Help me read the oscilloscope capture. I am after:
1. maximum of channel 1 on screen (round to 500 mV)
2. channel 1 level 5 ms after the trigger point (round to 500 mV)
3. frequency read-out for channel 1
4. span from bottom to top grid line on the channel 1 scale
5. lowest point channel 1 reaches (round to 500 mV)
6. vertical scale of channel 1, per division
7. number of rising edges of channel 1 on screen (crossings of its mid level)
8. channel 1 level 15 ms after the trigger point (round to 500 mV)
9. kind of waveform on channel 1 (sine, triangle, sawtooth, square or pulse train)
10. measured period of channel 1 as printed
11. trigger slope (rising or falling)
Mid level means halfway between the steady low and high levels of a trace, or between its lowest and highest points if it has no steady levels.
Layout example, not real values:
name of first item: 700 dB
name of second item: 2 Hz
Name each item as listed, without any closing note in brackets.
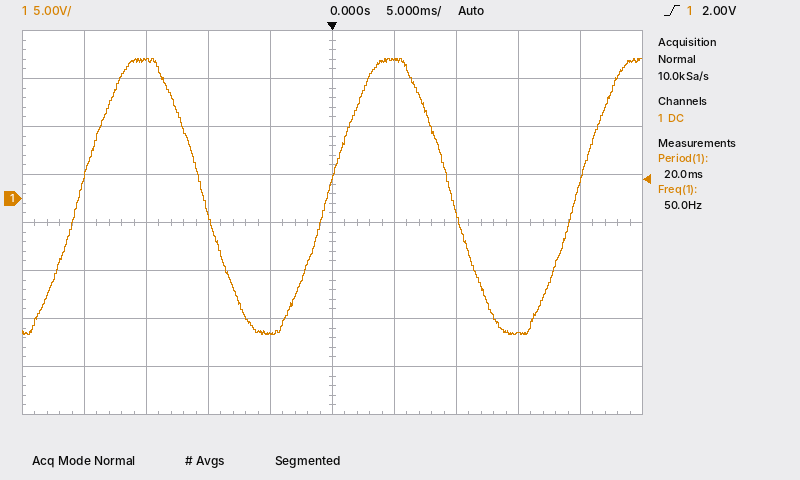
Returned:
maximum of channel 1 on screen: 14.5 V
channel 1 level 5 ms after the trigger point: 14.5 V
frequency read-out for channel 1: 50.0 Hz
span from bottom to top grid line on the channel 1 scale: 40 V
lowest point channel 1 reaches: -14.0 V
vertical scale of channel 1, per division: 5 V
number of rising edges of channel 1 on screen: 3
channel 1 level 15 ms after the trigger point: -14.0 V
kind of waveform on channel 1: sine
measured period of channel 1 as printed: 20.0 ms
trigger slope: rising
